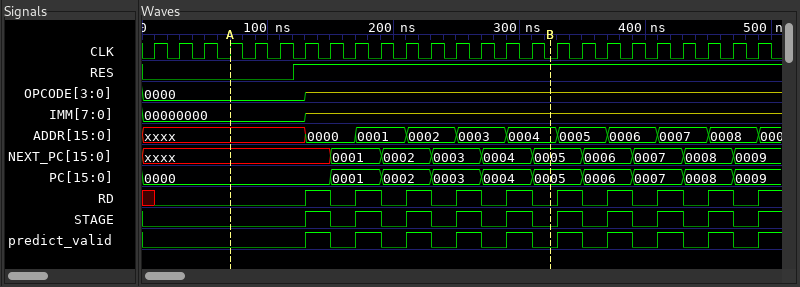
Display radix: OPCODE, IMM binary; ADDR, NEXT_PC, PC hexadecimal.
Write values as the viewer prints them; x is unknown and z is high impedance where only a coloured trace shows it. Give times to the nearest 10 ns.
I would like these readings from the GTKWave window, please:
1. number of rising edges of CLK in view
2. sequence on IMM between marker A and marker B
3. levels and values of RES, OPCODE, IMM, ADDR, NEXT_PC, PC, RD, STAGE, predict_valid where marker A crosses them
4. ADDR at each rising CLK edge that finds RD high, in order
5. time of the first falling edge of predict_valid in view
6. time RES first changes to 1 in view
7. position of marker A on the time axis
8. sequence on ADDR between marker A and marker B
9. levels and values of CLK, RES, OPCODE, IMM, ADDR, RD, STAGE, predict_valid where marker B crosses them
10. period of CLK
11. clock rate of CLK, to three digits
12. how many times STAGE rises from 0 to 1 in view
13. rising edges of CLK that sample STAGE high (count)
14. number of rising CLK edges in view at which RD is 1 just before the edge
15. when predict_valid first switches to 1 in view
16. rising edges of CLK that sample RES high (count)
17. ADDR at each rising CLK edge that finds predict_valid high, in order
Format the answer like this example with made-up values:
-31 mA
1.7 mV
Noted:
25
00000000, z
RES=0, OPCODE=0000, IMM=00000000, ADDR=xxxx, NEXT_PC=xxxx, PC=0000, RD=0, STAGE=0, predict_valid=0
0000, 0001, 0002, 0003, 0004, 0005, 0006, 0007, 0008
150 ns
120 ns
70 ns
xxxx, 0000, 0001, 0002, 0003, 0004
CLK=0, RES=1, OPCODE=z, IMM=z, ADDR=0004, RD=0, STAGE=0, predict_valid=0
20 ns
50.0 MHz
10
9
9
130 ns
19
0000, 0001, 0002, 0003, 0004, 0005, 0006, 0007, 0008
